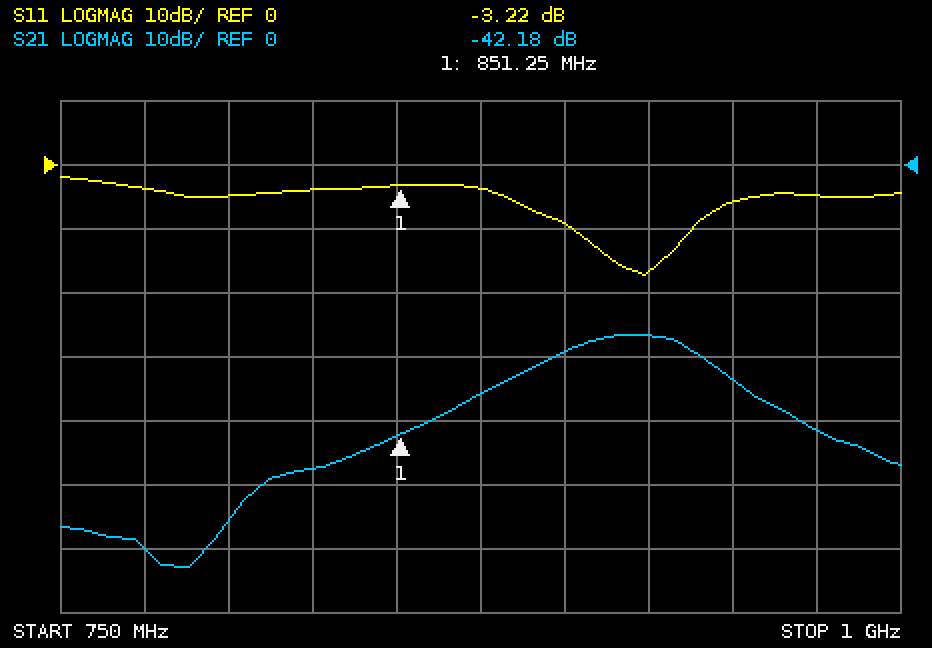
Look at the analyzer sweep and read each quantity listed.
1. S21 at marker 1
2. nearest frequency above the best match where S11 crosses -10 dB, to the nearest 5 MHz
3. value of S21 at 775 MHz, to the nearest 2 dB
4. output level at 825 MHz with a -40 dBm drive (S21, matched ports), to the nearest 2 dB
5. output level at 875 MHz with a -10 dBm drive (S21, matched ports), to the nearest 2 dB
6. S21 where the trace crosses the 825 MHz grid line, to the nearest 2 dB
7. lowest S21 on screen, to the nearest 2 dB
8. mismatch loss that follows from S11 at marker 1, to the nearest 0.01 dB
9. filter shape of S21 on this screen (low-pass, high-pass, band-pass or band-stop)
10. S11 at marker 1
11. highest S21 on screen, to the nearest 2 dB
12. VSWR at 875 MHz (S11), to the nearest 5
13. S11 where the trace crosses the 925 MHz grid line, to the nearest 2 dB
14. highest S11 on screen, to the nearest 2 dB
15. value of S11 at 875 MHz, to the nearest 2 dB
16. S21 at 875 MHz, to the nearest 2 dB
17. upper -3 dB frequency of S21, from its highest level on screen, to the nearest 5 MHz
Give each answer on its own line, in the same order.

-42.18 dB
940 MHz
-60 dB
-88 dBm
-46 dBm
-48 dB
-62 dB
2.81 dB
band-pass
-3.22 dB
-26 dB
5
-16 dB
-2 dB
-4 dB
-36 dB
940 MHz
